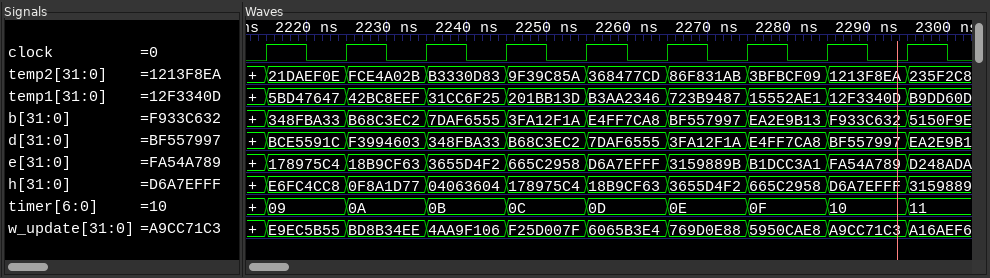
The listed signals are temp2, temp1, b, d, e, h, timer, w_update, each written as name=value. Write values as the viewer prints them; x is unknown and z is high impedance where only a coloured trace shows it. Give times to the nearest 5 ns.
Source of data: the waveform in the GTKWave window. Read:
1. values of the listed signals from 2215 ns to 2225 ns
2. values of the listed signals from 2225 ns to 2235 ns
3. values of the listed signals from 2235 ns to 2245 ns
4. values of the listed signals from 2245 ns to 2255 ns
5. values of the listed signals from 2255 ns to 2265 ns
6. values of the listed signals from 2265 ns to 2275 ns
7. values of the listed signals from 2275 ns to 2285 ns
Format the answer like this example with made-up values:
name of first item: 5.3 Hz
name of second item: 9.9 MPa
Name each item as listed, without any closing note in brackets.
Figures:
values of the listed signals from 2215 ns to 2225 ns: temp2=21DAEF0E, temp1=5BD47647, b=348FBA33, d=BCE5591C, e=178975C4, h=E6FC4CC8, timer=09, w_update=E9EC5B55
values of the listed signals from 2225 ns to 2235 ns: temp2=FCE4A02B, temp1=42BC8EEF, b=B68C3EC2, d=F3994603, e=18B9CF63, h=0F8A1D77, timer=0A, w_update=BD8B34EE
values of the listed signals from 2235 ns to 2245 ns: temp2=B3330D83, temp1=31CC6F25, b=7DAF6555, d=348FBA33, e=3655D4F2, h=04063604, timer=0B, w_update=4AA9F106
values of the listed signals from 2245 ns to 2255 ns: temp2=9F39C85A, temp1=201BB13D, b=3FA12F1A, d=B68C3EC2, e=665C2958, h=178975C4, timer=0C, w_update=F25D007F
values of the listed signals from 2255 ns to 2265 ns: temp2=368477CD, temp1=B3AA2346, b=E4FF7CA8, d=7DAF6555, e=D6A7EFFF, h=18B9CF63, timer=0D, w_update=6065B3E4
values of the listed signals from 2265 ns to 2275 ns: temp2=86F831AB, temp1=723B9487, b=BF557997, d=3FA12F1A, e=3159889B, h=3655D4F2, timer=0E, w_update=769D0E88
values of the listed signals from 2275 ns to 2285 ns: temp2=3BFBCF09, temp1=15552AE1, b=EA2E9B13, d=E4FF7CA8, e=B1DCC3A1, h=665C2958, timer=0F, w_update=5950CAE8
